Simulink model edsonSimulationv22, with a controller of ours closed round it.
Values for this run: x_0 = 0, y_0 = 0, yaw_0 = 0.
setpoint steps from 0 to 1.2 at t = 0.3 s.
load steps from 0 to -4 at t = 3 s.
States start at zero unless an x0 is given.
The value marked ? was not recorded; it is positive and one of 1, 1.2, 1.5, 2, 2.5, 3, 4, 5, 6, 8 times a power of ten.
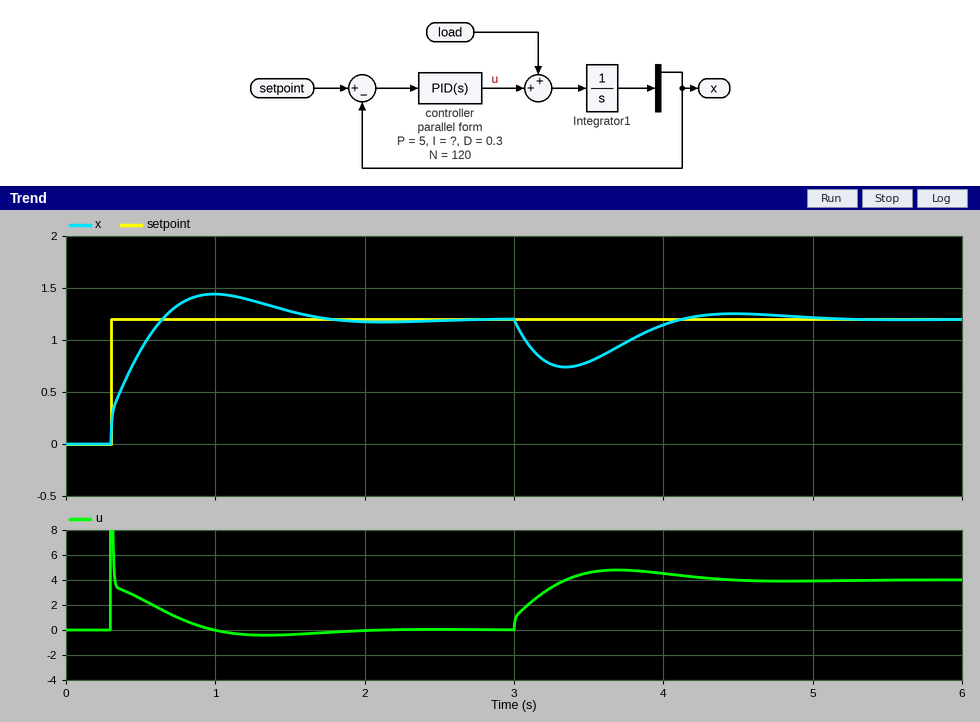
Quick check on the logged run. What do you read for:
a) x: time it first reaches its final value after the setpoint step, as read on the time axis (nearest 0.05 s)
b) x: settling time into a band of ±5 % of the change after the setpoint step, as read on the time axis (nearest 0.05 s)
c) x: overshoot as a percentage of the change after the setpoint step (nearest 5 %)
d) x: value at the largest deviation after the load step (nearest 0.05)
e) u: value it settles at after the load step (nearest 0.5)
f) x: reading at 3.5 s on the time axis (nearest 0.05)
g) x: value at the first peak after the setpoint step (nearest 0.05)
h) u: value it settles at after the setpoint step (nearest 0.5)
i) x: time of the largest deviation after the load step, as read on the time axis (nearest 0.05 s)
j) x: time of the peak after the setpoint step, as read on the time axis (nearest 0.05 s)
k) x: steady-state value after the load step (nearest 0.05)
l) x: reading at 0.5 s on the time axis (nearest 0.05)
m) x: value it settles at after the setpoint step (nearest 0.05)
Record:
0.65 s
1.55 s
20 %
0.75
4.0
0.80
1.45
0.0
3.35 s
1.00 s
1.20
0.90
1.20
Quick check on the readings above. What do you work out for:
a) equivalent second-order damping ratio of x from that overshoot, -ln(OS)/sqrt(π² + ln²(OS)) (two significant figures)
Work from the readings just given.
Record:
0.46
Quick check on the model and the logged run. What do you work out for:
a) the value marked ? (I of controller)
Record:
15
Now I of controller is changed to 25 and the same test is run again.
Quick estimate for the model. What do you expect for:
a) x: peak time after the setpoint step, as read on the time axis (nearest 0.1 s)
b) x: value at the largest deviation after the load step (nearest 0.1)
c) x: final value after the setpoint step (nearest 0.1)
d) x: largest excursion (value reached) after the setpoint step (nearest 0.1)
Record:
0.9 s
0.8
1.2
1.5
